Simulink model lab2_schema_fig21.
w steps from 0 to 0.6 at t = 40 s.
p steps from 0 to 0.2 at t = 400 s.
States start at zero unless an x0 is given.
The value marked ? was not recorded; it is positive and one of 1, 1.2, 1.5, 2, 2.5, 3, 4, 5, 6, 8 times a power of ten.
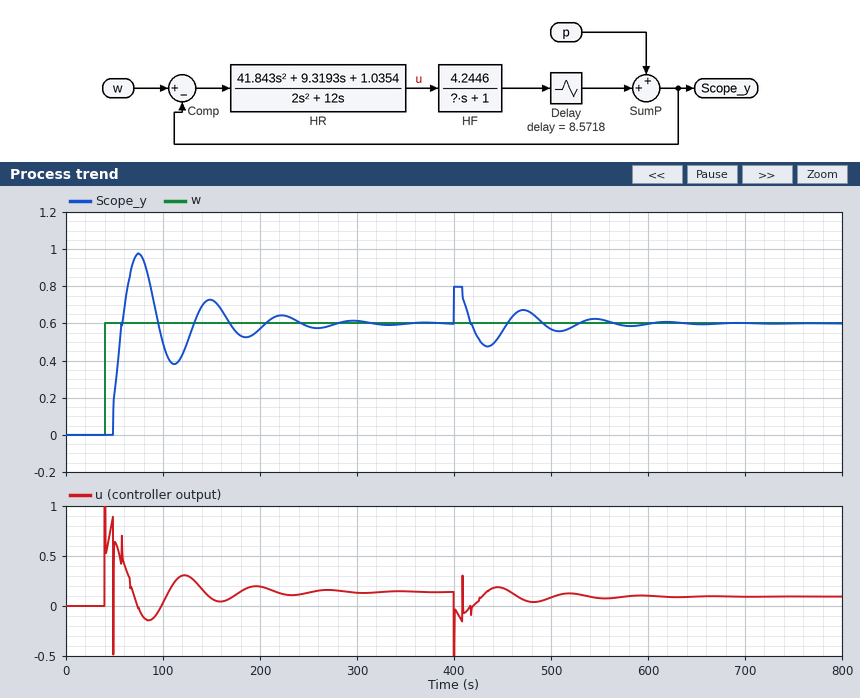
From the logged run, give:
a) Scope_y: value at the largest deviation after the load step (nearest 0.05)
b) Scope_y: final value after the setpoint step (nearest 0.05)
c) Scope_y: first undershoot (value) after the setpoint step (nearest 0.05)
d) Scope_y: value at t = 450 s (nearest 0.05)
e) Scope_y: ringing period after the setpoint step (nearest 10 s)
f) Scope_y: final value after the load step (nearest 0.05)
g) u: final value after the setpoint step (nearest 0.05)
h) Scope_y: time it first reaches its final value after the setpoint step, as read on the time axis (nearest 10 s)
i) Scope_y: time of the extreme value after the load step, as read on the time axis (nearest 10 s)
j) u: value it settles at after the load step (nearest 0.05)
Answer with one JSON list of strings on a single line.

["0.80", "0.60", "0.40", "0.55", "70 s", "0.60", "0.15", "60 s", "400 s", "0.10"]
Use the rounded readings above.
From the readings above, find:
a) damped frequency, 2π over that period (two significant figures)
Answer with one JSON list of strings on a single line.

["0.090 rad/s"]
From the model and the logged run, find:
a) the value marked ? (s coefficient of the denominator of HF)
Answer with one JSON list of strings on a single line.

["50"]
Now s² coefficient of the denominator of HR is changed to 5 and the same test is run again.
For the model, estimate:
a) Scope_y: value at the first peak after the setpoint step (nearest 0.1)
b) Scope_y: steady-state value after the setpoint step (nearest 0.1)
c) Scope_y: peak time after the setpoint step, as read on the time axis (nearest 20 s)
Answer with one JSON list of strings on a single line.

["1.0", "0.6", "80 s"]
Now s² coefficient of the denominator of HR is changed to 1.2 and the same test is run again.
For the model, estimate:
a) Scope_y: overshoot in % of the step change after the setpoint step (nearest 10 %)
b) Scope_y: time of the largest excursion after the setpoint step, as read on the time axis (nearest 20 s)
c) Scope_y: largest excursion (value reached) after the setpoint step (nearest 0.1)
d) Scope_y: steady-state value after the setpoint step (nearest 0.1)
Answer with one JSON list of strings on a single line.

["60 %", "80 s", "1.0", "0.6"]
